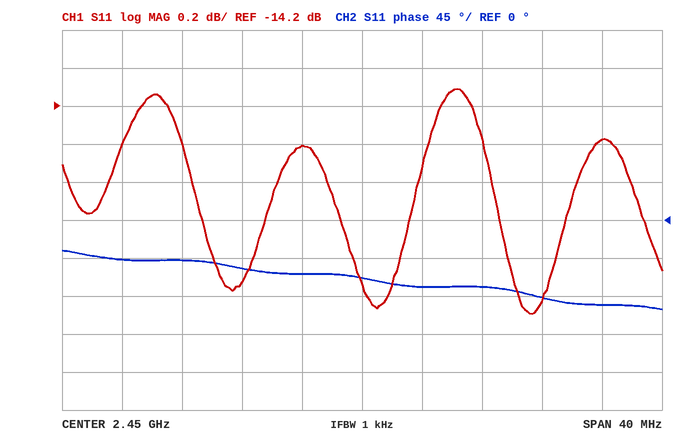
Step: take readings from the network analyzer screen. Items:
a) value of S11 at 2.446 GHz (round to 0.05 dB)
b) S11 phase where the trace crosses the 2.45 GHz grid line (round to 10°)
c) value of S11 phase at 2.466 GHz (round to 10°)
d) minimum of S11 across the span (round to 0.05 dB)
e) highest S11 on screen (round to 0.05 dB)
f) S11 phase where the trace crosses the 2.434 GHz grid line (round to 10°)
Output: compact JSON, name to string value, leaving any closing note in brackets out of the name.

{"value of S11 at 2.446 GHz": "-14.40 dB", "S11 phase where the trace crosses the 2.45 GHz grid line": "-70°", "value of S11 phase at 2.466 GHz": "-100°", "minimum of S11 across the span": "-15.30 dB", "highest S11 on screen": "-14.10 dB", "S11 phase where the trace crosses the 2.434 GHz grid line": "-50°"}
